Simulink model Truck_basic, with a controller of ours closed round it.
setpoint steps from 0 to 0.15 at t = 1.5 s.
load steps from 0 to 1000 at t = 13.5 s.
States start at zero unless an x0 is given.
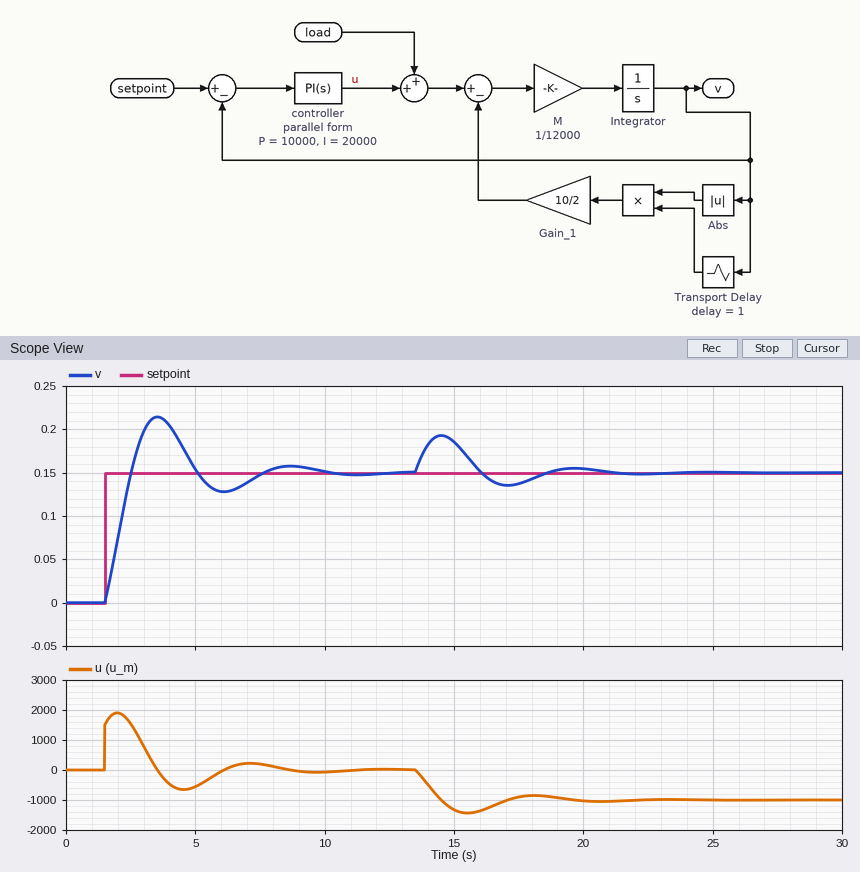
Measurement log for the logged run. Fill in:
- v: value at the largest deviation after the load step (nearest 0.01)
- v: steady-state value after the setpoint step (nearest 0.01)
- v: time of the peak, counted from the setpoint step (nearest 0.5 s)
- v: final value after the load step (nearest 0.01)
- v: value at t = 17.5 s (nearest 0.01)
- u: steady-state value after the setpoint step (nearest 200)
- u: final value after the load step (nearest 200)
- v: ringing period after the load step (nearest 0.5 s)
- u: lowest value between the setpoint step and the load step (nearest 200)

0.19
0.15
2.0 s
0.15
0.14
0
-1000
5.0 s
-600
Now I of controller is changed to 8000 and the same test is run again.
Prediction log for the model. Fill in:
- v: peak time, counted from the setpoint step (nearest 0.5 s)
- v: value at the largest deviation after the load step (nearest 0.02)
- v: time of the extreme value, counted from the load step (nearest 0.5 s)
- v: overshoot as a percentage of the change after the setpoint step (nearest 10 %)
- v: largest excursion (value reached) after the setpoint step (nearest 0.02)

3.0 s
0.20
1.5 s
30 %
0.20
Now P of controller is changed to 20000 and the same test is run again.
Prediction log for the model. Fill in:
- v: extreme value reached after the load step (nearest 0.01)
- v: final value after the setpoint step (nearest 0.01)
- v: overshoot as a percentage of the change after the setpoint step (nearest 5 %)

0.18
0.15
25 %
